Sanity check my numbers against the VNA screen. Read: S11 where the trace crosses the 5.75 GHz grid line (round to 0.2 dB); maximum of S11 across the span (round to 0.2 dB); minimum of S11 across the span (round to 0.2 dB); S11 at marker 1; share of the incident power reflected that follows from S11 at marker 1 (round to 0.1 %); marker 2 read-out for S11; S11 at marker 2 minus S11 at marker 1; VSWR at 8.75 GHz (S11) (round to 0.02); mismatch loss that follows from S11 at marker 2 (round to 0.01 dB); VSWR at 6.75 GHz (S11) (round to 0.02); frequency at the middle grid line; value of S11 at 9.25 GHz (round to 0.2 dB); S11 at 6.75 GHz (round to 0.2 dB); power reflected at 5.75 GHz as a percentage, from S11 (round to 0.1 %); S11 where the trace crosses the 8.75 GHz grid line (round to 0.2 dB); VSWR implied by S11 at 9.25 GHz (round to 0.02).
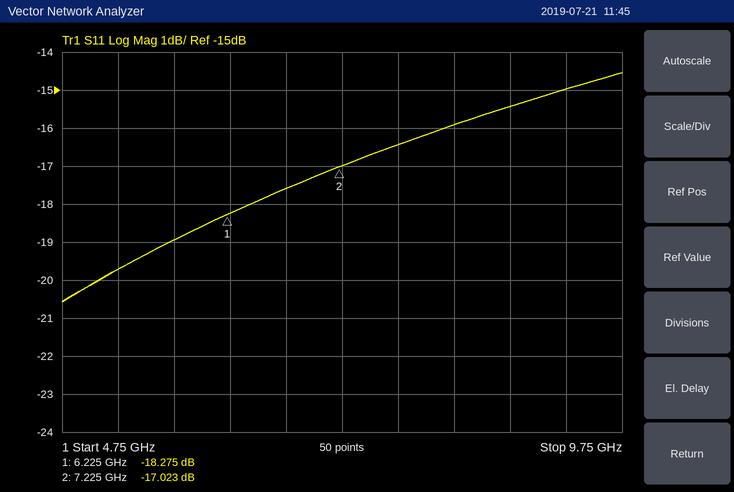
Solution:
-19.0 dB
-14.6 dB
-20.6 dB
-18.275 dB
1.5 %
-17.023 dB
1.252 dB
1.40
0.09 dB
1.30
7.25 GHz
-15.0 dB
-17.6 dB
1.3 %
-15.4 dB
1.44
